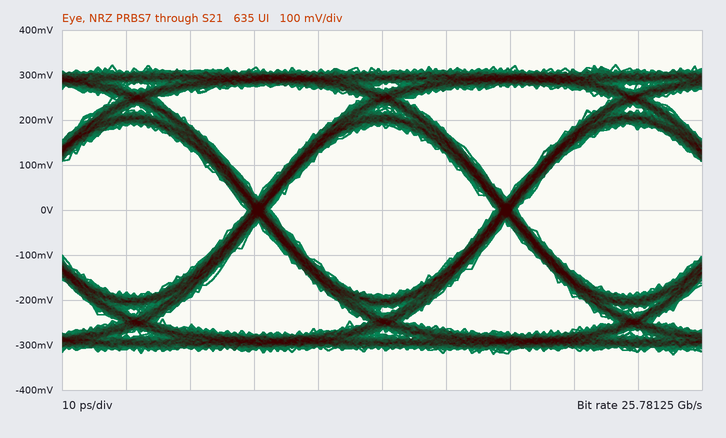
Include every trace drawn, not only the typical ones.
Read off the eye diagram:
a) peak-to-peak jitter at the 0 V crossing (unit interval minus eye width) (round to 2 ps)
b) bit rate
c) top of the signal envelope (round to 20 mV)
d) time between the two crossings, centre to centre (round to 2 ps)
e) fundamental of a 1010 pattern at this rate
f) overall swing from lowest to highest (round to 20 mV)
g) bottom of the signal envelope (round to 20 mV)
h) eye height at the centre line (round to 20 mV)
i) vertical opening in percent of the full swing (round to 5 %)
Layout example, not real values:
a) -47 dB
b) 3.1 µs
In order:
a) 4 ps
b) 25.78125 Gb/s
c) 320 mV
d) 38 ps
e) 12.89062 GHz
f) 640 mV
g) -320 mV
h) 380 mV
i) 60 %
